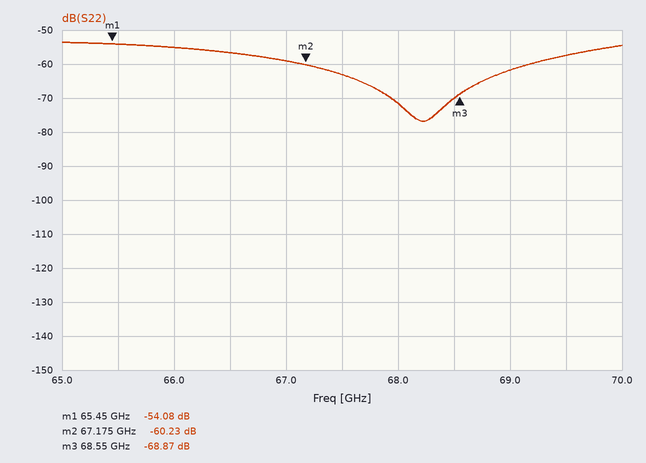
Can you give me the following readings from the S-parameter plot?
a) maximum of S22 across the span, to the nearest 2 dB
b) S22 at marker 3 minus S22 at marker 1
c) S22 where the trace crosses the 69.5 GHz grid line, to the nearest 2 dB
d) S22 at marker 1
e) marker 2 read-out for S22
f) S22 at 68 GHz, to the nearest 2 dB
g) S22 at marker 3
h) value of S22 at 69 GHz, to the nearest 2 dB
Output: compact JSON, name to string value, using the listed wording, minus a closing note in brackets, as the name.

{"maximum of S22 across the span, to the nearest 2 dB": "-54 dB", "S22 at marker 3 minus S22 at marker 1": "-14.79 dB", "S22 where the trace crosses the 69.5 GHz grid line, to the nearest 2 dB": "-58 dB", "S22 at marker 1": "-54.08 dB", "marker 2 read-out for S22": "-60.23 dB", "S22 at 68 GHz, to the nearest 2 dB": "-72 dB", "S22 at marker 3": "-68.87 dB", "value of S22 at 69 GHz, to the nearest 2 dB": "-62 dB"}
